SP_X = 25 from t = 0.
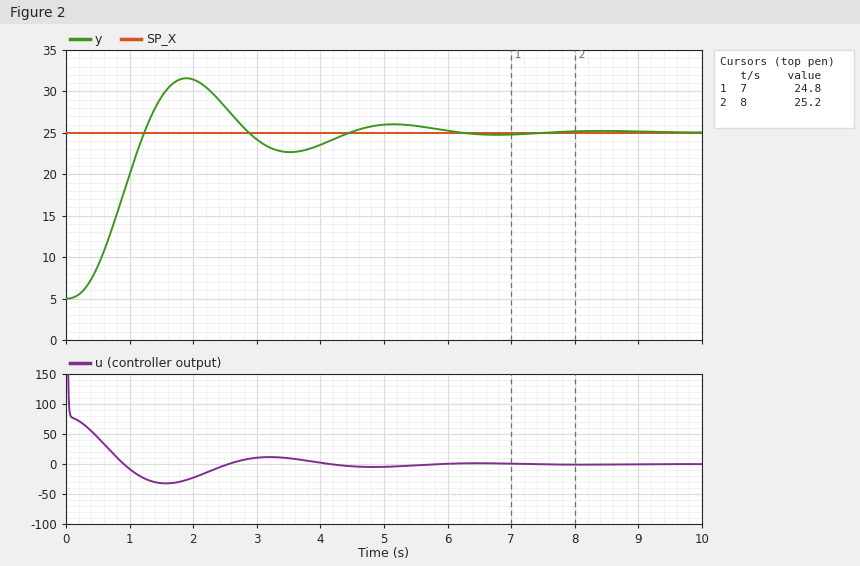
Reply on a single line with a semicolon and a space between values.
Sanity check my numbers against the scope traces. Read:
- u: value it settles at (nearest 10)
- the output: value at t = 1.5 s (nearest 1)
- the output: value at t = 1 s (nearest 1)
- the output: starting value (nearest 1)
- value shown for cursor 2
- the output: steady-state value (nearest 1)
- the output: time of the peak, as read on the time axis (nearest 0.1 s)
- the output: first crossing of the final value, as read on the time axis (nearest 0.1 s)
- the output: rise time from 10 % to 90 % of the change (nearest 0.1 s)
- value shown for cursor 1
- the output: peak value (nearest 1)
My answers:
0; 29; 20; 5; 25.2; 25; 1.9 s; 1.2 s; 0.8 s; 24.8; 32
